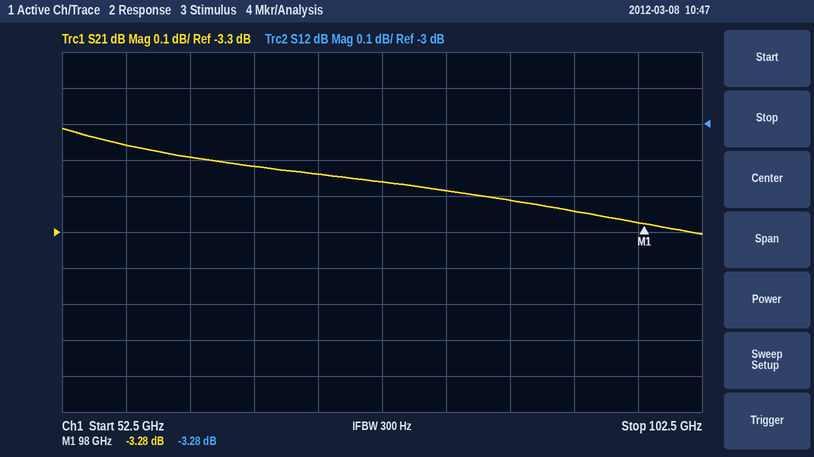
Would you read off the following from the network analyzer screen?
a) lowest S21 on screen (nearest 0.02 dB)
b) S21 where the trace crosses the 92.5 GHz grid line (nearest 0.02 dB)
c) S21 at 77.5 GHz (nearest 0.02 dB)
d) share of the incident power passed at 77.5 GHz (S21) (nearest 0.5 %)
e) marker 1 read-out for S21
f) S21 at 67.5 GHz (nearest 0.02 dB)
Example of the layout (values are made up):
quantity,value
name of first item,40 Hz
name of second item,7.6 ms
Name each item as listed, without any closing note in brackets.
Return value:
quantity,value
lowest S21 on screen,-3.30 dB
S21 where the trace crosses the 92.5 GHz grid line,-3.24 dB
S21 at 77.5 GHz,-3.16 dB
share of the incident power passed at 77.5 GHz (S21),48.5 %
marker 1 read-out for S21,-3.28 dB
S21 at 67.5 GHz,-3.12 dB
